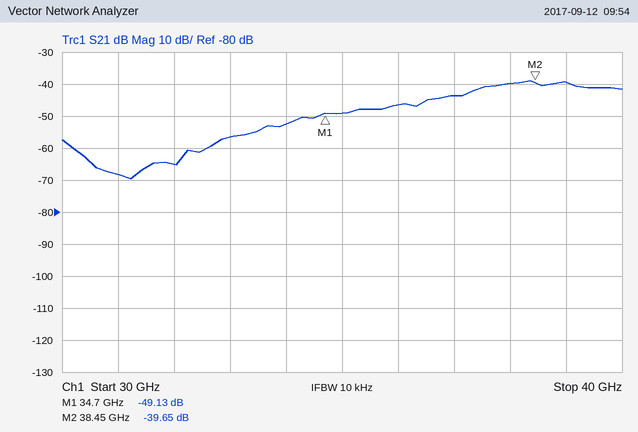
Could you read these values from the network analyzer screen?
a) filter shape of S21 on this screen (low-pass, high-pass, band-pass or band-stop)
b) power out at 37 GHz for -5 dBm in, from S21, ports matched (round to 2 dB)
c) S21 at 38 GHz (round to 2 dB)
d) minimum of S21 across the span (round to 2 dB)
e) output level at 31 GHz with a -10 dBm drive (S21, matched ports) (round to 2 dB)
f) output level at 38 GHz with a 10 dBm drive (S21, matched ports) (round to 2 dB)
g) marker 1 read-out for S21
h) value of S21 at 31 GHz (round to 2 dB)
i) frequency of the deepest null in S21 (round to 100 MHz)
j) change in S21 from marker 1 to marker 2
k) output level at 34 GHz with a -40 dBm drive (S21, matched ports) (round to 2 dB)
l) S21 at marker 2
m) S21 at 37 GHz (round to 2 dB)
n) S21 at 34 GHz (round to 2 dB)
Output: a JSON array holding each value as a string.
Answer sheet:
["high-pass", "-48 dBm", "-40 dB", "-70 dB", "-78 dBm", "-30 dBm", "-49.13 dB", "-68 dB", "31.2 GHz", "9.48 dB", "-92 dBm", "-39.65 dB", "-44 dB", "-52 dB"]
